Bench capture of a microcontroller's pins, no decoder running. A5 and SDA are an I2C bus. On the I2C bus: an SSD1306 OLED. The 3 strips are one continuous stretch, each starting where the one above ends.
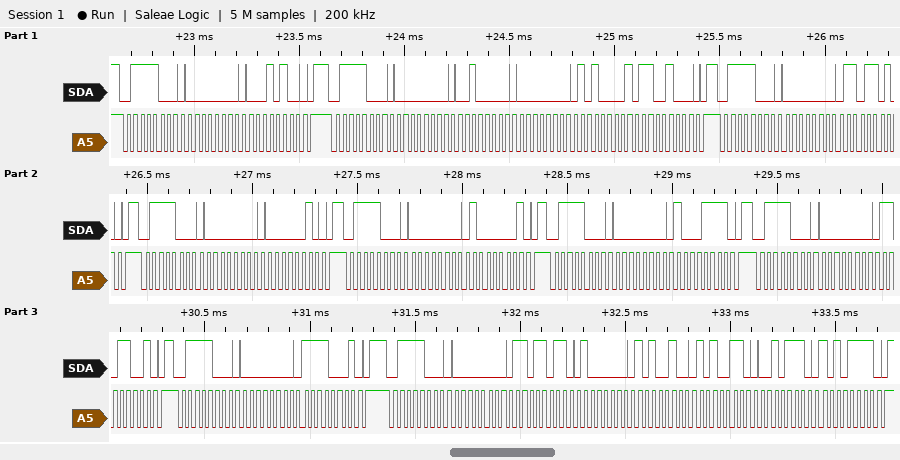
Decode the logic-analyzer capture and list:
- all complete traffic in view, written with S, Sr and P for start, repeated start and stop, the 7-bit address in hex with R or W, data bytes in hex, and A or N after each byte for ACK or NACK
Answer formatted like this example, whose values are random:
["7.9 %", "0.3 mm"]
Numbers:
["S 3CW A 00 A 14 A P S 3CW A 00 A 20 A 00 A A1 A C8 A P S 3CW A 00 A DA A P S 3CW A 00 A 02 A P S 3CW A 00 A 81 A P S 3CW A 00 A 8F A P S 3CW A 00 A D9 A P S 3CW A 00 A F1 A P S 3CW A 00 A DB A 40 A A4 A A6 A 2E A AF A P"]
